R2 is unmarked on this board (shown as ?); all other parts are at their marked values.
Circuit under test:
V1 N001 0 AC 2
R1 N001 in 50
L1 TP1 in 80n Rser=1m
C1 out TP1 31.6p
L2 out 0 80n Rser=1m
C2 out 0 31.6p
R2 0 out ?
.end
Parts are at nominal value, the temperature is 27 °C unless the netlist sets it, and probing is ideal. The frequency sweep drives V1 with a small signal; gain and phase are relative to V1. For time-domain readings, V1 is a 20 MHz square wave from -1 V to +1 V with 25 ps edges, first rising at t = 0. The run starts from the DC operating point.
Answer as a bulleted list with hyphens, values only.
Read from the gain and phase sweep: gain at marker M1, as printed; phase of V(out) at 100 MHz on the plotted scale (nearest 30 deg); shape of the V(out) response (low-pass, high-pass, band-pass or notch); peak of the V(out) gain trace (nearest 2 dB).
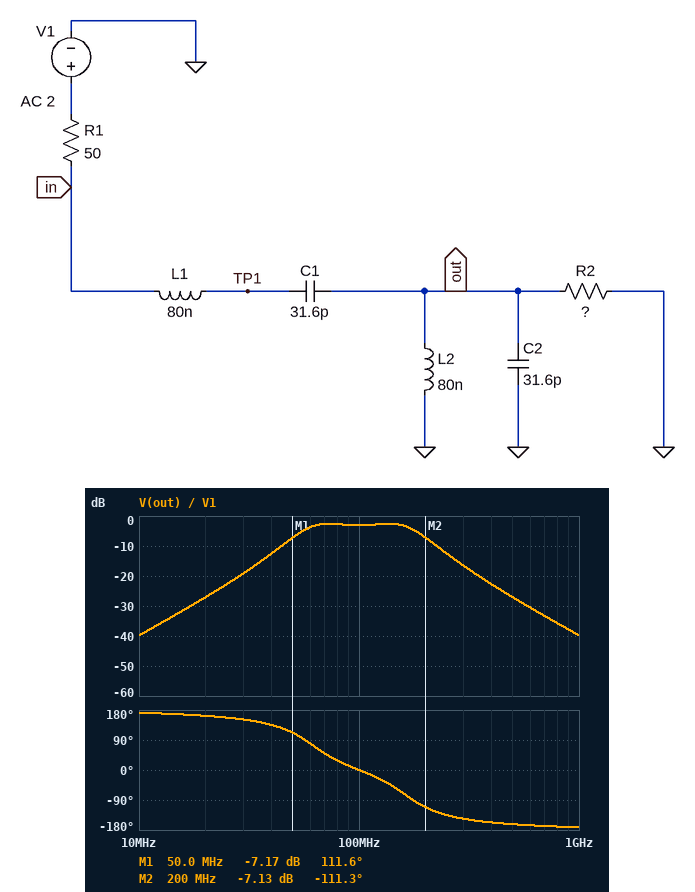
- -7.17 dB
- 0 deg
- band-pass
- -2 dB
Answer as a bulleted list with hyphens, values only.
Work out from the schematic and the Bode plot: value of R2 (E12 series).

- 120 Ω
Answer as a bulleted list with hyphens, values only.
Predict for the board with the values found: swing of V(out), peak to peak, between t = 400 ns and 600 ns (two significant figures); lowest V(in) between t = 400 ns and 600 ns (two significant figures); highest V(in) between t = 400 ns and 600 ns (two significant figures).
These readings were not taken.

- 1.3 V
- -1.2 V
- 1.2 V
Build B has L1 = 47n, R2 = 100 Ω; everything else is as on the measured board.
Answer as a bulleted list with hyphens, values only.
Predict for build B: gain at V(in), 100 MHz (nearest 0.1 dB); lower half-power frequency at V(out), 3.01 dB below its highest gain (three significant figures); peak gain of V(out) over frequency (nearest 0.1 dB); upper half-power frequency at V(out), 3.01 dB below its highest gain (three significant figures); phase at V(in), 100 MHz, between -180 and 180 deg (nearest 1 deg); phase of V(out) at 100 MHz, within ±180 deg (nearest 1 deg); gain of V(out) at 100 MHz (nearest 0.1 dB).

- -3.4 dB
- 55.6 MHz
- -3.0 dB
- 210 MHz
- -4 deg
- 8 deg
- -3.6 dB
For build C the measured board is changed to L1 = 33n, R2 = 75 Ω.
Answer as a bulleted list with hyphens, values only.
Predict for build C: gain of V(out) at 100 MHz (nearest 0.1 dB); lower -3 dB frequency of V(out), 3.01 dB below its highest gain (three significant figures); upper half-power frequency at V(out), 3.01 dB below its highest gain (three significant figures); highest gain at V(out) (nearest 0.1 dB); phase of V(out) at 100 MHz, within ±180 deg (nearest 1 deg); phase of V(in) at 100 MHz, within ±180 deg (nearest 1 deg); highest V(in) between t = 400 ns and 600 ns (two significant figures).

- -4.7 dB
- 55.4 MHz
- 232 MHz
- -4.3 dB
- 13 deg
- -8 deg
- 1.1 V
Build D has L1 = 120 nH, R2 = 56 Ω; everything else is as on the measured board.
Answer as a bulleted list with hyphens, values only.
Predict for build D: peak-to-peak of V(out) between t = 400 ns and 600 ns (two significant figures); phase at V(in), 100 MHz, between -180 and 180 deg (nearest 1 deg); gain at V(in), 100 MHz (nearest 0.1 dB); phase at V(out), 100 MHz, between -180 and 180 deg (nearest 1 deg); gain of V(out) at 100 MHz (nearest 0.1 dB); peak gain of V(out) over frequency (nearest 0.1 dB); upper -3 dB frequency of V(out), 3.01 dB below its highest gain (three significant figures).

- 950 mV
- 11 deg
- -5.0 dB
- -13 deg
- -5.8 dB
- -5.7 dB
- 166 MHz
